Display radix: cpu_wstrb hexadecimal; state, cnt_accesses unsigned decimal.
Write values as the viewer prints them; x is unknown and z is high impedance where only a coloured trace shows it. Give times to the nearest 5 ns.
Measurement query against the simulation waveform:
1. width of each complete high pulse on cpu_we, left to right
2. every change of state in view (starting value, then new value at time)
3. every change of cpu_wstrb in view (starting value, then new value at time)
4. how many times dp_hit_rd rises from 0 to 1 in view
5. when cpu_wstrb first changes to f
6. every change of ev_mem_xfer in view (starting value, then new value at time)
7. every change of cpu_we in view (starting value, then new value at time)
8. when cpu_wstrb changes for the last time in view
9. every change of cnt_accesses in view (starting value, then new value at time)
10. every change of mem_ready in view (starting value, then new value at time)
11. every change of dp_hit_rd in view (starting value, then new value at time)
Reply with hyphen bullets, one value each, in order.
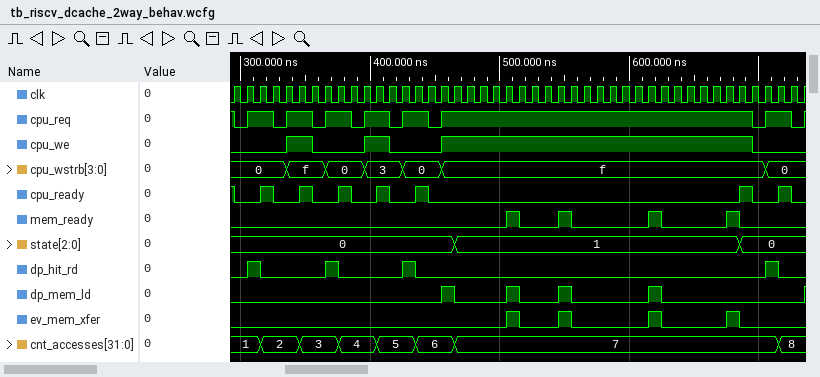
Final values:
- 20 ns, 20 ns, 240 ns
- 0, 1 at 465 ns, 0 at 685 ns
- 0, f at 335 ns, 0 at 365 ns, 3 at 395 ns, 0 at 425 ns, f at 455 ns, 0 at 705 ns
- 4
- 335 ns
- 0, 1 at 505 ns, 0 at 515 ns, 1 at 545 ns, 0 at 555 ns, 1 at 615 ns, 0 at 625 ns, 1 at 675 ns, 0 at 685 ns
- 0, 1 at 335 ns, 0 at 355 ns, 1 at 395 ns, 0 at 415 ns, 1 at 455 ns, 0 at 695 ns
- 705 ns
- 1, 2 at 315 ns, 3 at 345 ns, 4 at 375 ns, 5 at 405 ns, 6 at 435 ns, 7 at 465 ns, 8 at 715 ns
- 0, 1 at 505 ns, 0 at 515 ns, 1 at 545 ns, 0 at 555 ns, 1 at 615 ns, 0 at 625 ns, 1 at 675 ns, 0 at 685 ns
- 0, 1 at 305 ns, 0 at 315 ns, 1 at 365 ns, 0 at 375 ns, 1 at 425 ns, 0 at 435 ns, 1 at 705 ns, 0 at 715 ns
